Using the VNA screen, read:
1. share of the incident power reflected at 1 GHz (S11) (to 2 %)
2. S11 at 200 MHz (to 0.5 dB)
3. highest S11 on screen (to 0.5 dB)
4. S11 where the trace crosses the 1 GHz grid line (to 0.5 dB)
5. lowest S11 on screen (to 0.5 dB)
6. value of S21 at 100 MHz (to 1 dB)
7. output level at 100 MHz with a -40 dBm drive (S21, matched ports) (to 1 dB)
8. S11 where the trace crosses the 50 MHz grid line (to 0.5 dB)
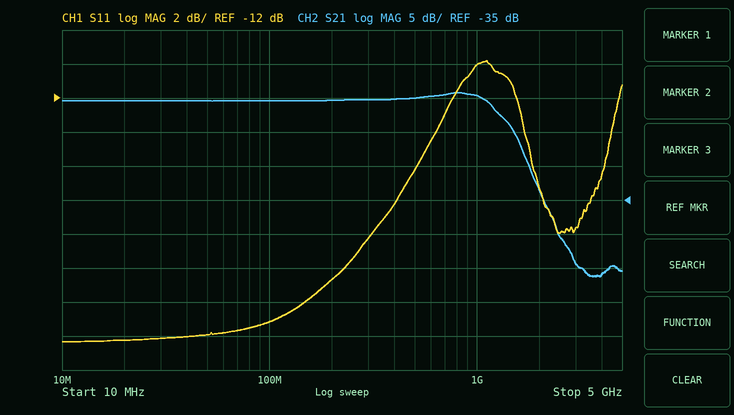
10 %
-22.5 dB
-10.0 dB
-10.0 dB
-26.5 dB
-20 dB
-60 dBm
-26.0 dB
